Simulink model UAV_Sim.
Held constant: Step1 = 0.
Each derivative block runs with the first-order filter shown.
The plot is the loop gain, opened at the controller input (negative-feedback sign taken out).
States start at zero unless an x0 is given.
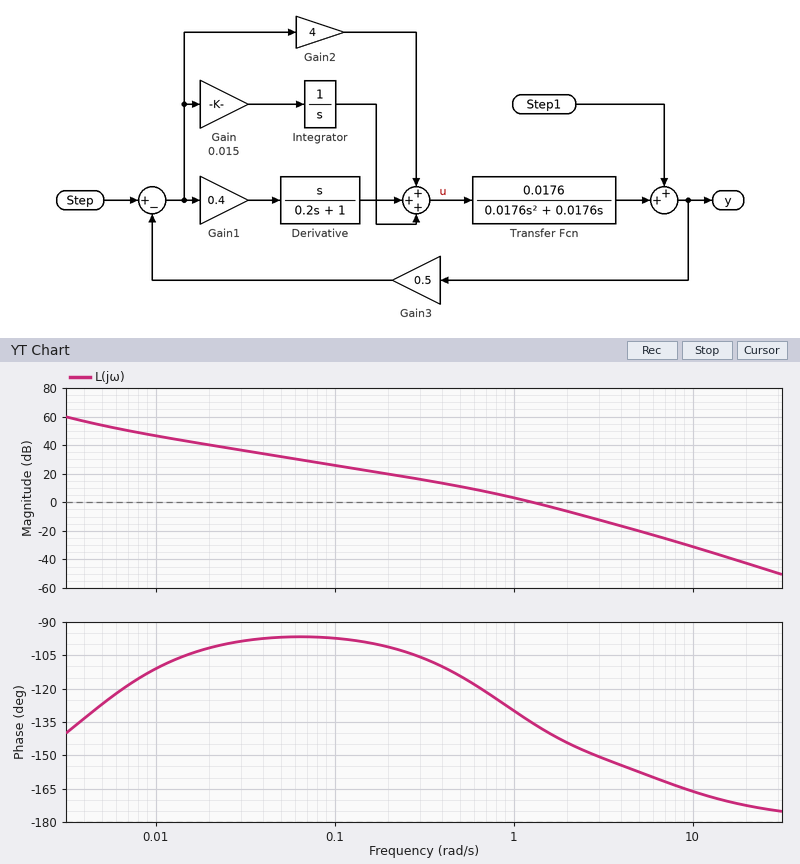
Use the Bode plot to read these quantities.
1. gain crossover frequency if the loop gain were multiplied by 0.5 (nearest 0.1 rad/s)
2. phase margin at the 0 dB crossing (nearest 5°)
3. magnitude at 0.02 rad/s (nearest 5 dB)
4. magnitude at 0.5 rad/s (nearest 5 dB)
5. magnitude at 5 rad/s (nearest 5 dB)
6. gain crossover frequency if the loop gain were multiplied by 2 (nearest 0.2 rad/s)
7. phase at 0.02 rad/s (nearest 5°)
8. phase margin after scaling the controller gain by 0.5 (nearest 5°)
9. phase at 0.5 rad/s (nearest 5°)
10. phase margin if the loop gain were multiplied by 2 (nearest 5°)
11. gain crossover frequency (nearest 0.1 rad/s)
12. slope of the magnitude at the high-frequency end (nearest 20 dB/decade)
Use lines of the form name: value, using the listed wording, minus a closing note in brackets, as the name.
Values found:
gain crossover frequency if the loop gain were multiplied by 0.5: 0.8 rad/s
phase margin at the 0 dB crossing: 45°
magnitude at 0.02 rad/s: 40 dB
magnitude at 0.5 rad/s: 10 dB
magnitude at 5 rad/s: -20 dB
gain crossover frequency if the loop gain were multiplied by 2: 2.0 rad/s
phase at 0.02 rad/s: -100°
phase margin after scaling the controller gain by 0.5: 55°
phase at 0.5 rad/s: -115°
phase margin if the loop gain were multiplied by 2: 35°
gain crossover frequency: 1.3 rad/s
slope of the magnitude at the high-frequency end: -40 dB/decade
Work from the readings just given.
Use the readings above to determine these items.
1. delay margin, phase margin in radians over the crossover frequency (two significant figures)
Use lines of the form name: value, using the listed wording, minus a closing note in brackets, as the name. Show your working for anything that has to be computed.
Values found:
delay margin, phase margin in radians over the crossover frequency: 45 × π / 180 / 1.3 = 0.60 s
